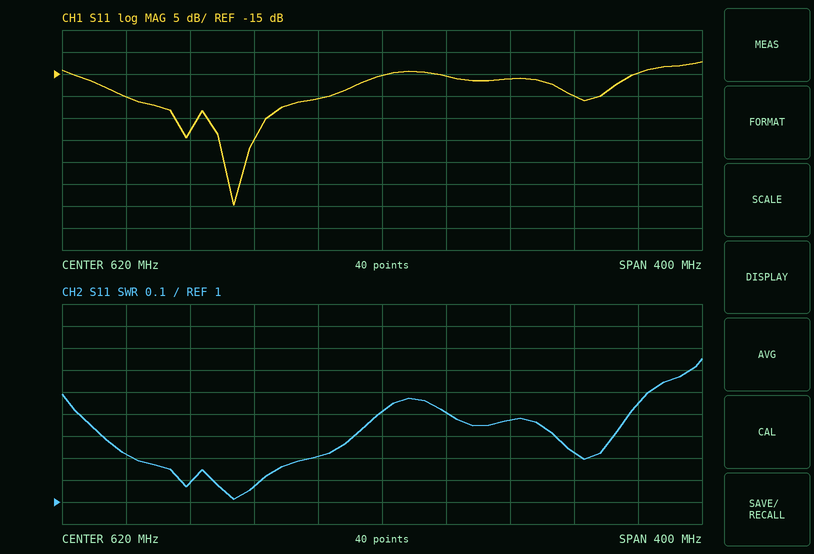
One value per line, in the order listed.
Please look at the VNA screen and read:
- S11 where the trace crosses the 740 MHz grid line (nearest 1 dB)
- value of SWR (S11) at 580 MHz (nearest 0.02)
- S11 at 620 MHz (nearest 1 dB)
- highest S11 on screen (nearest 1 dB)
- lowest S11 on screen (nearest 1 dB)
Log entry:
-20 dB
1.20
-15 dB
-12 dB
-45 dB
